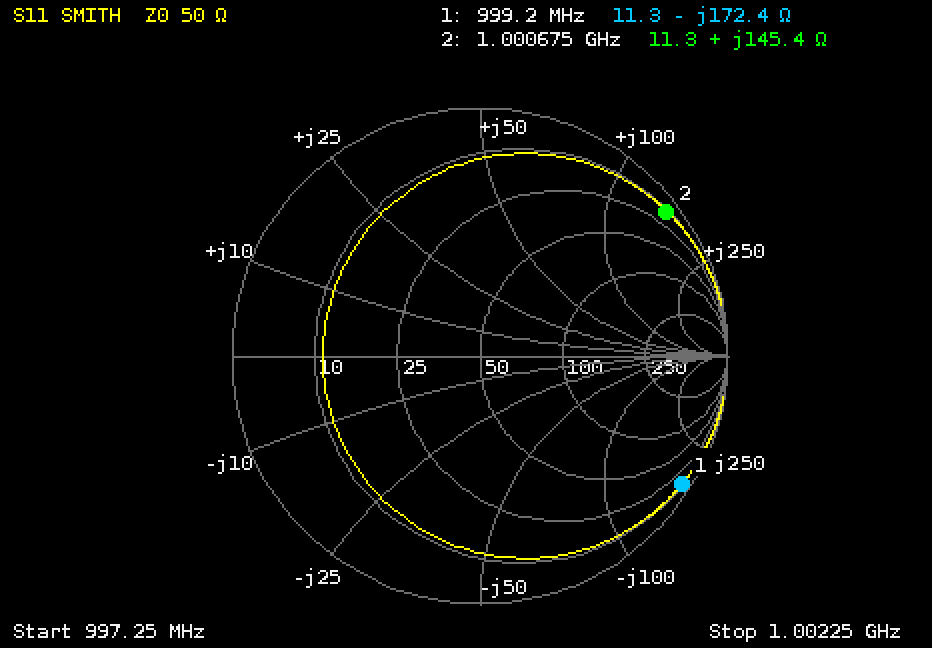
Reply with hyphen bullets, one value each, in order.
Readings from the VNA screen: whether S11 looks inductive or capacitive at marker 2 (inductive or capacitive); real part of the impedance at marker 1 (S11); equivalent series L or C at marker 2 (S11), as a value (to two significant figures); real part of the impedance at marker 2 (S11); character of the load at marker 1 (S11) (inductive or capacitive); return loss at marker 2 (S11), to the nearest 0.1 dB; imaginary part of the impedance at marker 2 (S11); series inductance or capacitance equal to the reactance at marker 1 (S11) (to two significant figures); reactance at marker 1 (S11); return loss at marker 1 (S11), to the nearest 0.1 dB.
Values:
- inductive
- 11.3 Ω
- 23 nH
- 11.3 Ω
- capacitive
- 0.4 dB
- +145.4 Ω
- 920 fF
- -172.4 Ω
- 0.3 dB
